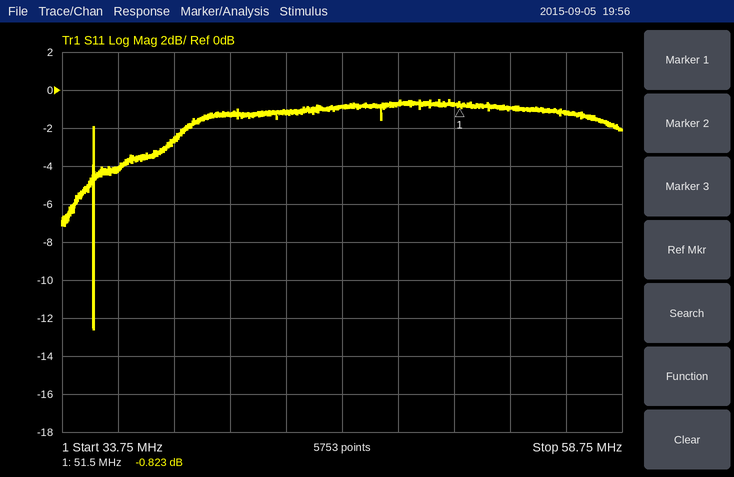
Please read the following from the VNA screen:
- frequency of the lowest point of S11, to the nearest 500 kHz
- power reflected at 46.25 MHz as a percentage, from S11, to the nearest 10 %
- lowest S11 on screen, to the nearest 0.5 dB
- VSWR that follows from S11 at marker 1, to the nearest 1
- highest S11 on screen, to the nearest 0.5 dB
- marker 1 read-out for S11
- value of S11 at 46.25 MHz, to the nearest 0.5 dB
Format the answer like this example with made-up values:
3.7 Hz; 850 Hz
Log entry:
35.0 MHz; 80 %; -12.5 dB; 21; -0.5 dB; -0.823 dB; -1.0 dB
